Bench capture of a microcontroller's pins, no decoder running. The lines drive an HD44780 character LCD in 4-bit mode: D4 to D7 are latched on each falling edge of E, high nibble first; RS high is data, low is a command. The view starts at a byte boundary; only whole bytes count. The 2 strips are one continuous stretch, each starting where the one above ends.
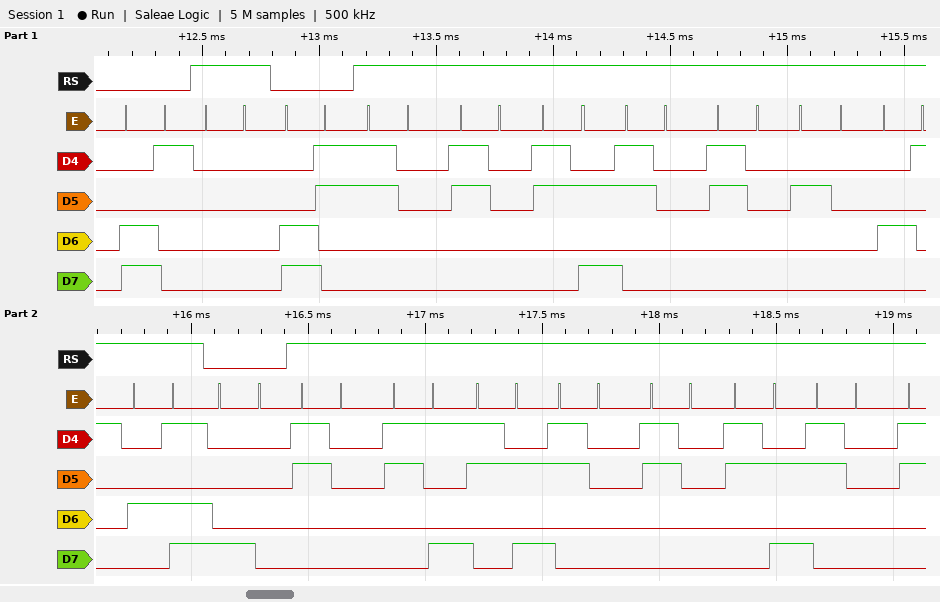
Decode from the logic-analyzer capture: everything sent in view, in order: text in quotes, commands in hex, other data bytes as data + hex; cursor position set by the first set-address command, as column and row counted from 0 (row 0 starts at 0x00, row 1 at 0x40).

0xC1 data 00 0xC3 "00:00 AM" 0x80 "09:00:0"
column 1, row 1
